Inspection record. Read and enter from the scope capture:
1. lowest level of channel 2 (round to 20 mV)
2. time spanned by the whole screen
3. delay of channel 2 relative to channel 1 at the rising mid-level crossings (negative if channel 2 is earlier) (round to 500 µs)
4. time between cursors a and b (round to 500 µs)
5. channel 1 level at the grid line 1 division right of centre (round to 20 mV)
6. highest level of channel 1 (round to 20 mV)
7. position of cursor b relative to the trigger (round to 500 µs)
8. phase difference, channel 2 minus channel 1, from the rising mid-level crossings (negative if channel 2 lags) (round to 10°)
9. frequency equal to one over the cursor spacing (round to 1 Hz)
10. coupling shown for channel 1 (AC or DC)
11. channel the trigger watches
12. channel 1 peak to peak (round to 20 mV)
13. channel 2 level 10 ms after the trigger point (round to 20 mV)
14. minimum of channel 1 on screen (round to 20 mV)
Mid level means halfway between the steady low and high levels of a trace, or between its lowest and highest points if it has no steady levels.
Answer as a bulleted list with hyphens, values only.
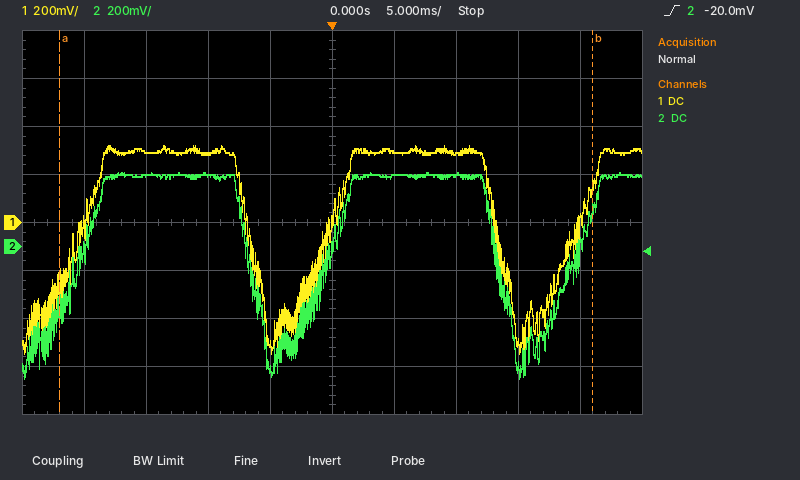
- -560 mV
- 50 ms
- 0.0 ms
- 43.0 ms
- 300 mV
- 320 mV
- +21.0 ms
- 0°
- 23 Hz
- DC
- channel 2
- 860 mV
- 300 mV
- -540 mV
